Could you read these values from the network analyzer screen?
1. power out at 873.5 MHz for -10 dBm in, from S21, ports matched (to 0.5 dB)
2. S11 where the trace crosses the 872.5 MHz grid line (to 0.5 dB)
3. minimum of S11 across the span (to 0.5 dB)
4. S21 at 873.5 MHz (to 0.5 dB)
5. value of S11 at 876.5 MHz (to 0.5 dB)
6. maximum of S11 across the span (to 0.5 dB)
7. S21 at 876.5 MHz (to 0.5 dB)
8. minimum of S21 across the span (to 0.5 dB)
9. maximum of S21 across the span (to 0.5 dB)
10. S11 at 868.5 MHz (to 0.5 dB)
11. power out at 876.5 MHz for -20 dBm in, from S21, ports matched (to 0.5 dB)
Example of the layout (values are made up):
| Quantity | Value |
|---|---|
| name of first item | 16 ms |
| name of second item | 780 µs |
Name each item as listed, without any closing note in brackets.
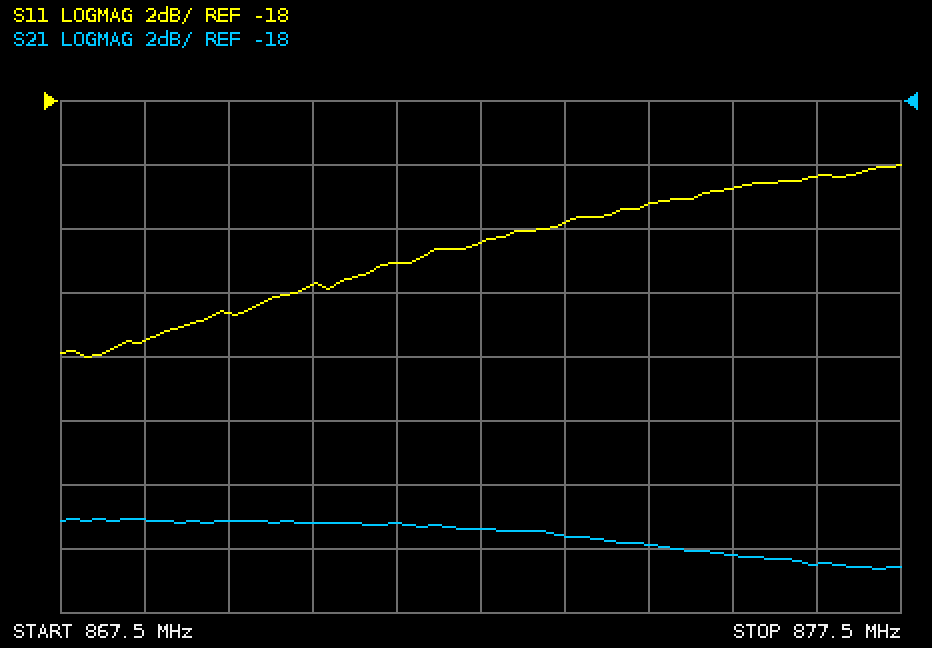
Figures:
| Quantity | Value |
|---|---|
| power out at 873.5 MHz for -10 dBm in, from S21, ports matched | -41.5 dBm |
| S11 where the trace crosses the 872.5 MHz grid line | -22.5 dB |
| minimum of S11 across the span | -26.0 dB |
| S21 at 873.5 MHz | -31.5 dB |
| value of S11 at 876.5 MHz | -20.5 dB |
| maximum of S11 across the span | -20.0 dB |
| S21 at 876.5 MHz | -32.5 dB |
| minimum of S21 across the span | -32.5 dB |
| maximum of S21 across the span | -31.0 dB |
| S11 at 868.5 MHz | -25.5 dB |
| power out at 876.5 MHz for -20 dBm in, from S21, ports matched | -52.5 dBm |
